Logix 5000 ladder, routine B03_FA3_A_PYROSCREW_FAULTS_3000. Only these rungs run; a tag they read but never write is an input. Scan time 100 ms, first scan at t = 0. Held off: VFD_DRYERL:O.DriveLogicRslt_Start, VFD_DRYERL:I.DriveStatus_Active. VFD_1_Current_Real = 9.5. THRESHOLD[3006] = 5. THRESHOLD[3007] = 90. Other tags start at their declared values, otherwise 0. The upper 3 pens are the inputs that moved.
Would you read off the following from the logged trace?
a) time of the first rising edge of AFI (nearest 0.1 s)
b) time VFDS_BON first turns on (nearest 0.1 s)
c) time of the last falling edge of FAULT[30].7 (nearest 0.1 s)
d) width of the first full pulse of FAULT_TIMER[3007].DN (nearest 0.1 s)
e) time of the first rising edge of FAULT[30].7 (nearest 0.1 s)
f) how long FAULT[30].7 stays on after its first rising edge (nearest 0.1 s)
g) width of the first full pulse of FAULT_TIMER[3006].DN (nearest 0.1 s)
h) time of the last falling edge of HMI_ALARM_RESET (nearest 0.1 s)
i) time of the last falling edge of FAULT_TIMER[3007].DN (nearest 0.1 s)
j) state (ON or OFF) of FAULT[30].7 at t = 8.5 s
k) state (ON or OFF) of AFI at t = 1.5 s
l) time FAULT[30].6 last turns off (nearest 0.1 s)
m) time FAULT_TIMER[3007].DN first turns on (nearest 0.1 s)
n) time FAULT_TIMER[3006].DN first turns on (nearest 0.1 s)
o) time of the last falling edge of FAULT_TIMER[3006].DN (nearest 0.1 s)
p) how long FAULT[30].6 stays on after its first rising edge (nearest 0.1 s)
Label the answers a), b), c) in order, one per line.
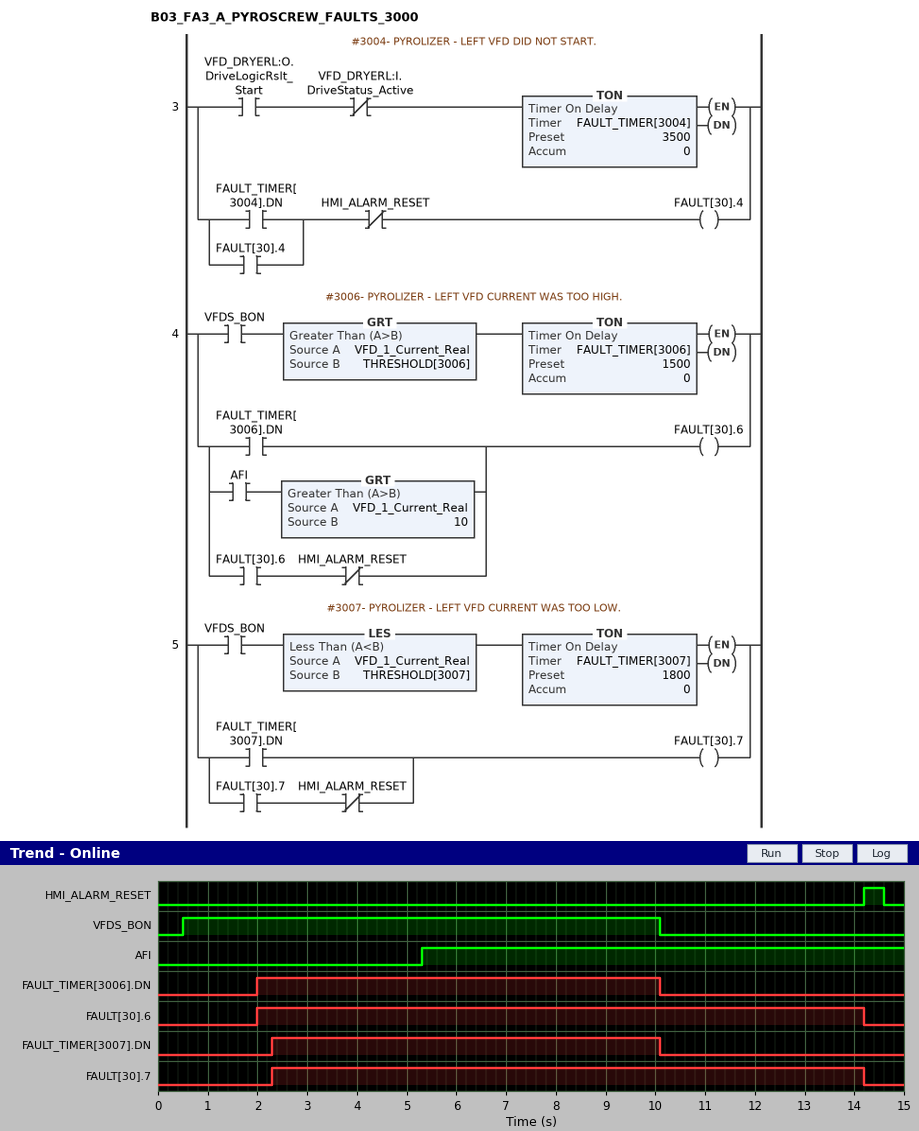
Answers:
a) 5.3 s
b) 0.5 s
c) 14.2 s
d) 7.8 s
e) 2.3 s
f) 11.9 s
g) 8.1 s
h) 14.6 s
i) 10.1 s
j) ON
k) OFF
l) 14.2 s
m) 2.3 s
n) 2.0 s
o) 10.1 s
p) 12.2 s
